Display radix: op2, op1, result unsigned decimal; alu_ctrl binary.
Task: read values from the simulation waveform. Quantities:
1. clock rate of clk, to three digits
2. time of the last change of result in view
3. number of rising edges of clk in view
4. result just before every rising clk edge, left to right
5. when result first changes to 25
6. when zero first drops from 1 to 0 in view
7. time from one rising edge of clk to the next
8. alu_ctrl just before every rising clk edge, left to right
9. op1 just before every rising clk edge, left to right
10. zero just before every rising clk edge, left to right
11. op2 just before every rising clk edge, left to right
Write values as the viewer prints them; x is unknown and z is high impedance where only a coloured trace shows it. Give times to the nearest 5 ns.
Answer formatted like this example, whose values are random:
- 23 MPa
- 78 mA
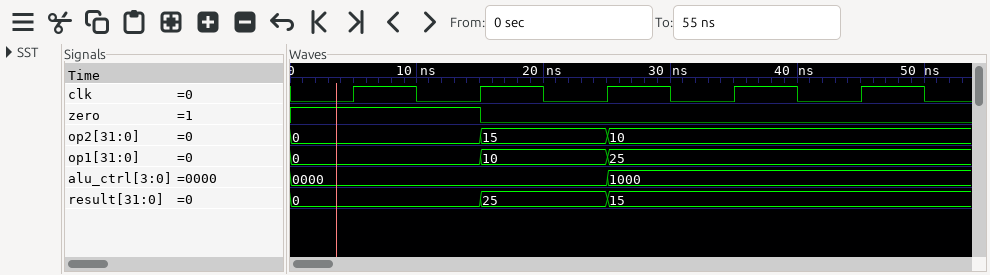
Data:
- 100 MHz
- 25 ns
- 5
- 0, 0, 25, 15, 15
- 15 ns
- 15 ns
- 10 ns
- 0000, 0000, 0000, 1000, 1000
- 0, 0, 10, 25, 25
- 1 1 0 0 0
- 0, 0, 15, 10, 10
